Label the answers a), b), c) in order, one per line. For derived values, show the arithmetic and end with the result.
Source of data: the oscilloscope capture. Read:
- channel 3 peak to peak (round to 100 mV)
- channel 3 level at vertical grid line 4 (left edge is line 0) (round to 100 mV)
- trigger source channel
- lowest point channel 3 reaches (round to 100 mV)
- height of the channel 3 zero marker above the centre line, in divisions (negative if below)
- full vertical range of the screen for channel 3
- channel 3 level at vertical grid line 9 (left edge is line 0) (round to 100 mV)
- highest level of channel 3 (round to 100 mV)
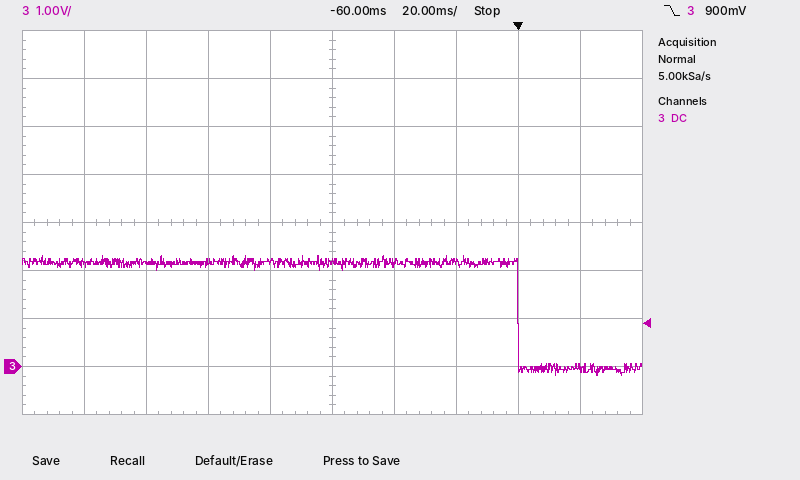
a) 2.3 V − (-200 mV) = 2.5 V
b) 2.2 V
c) channel 3
d) -200 mV
e) -3.0 div
f) 8 V
g) 0.0 V
h) 2.3 V
